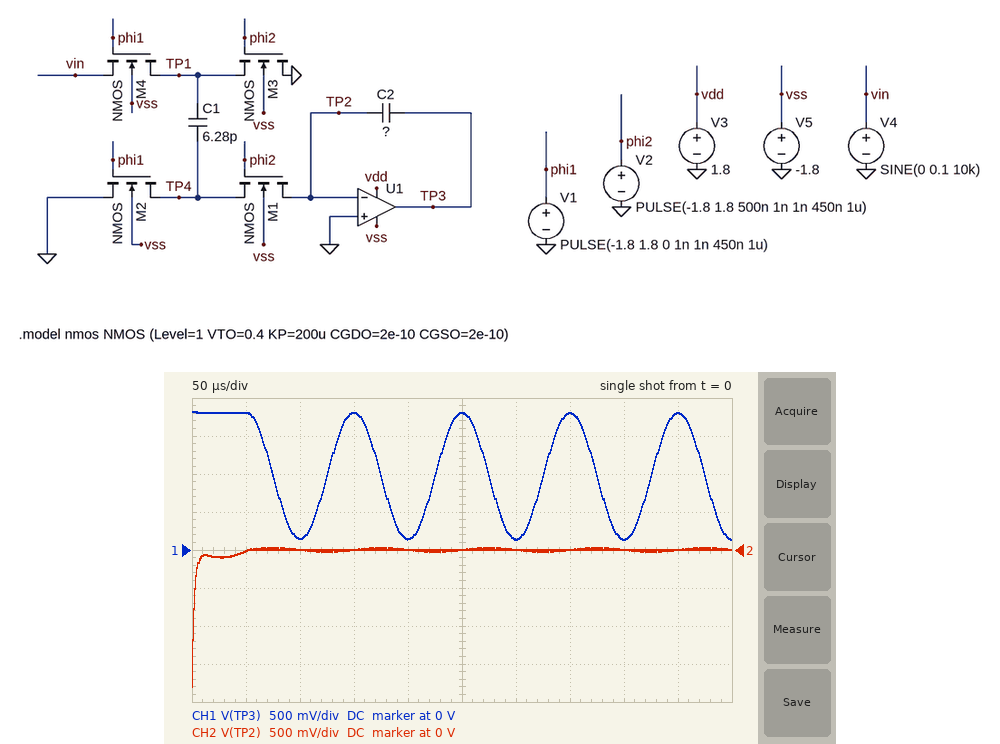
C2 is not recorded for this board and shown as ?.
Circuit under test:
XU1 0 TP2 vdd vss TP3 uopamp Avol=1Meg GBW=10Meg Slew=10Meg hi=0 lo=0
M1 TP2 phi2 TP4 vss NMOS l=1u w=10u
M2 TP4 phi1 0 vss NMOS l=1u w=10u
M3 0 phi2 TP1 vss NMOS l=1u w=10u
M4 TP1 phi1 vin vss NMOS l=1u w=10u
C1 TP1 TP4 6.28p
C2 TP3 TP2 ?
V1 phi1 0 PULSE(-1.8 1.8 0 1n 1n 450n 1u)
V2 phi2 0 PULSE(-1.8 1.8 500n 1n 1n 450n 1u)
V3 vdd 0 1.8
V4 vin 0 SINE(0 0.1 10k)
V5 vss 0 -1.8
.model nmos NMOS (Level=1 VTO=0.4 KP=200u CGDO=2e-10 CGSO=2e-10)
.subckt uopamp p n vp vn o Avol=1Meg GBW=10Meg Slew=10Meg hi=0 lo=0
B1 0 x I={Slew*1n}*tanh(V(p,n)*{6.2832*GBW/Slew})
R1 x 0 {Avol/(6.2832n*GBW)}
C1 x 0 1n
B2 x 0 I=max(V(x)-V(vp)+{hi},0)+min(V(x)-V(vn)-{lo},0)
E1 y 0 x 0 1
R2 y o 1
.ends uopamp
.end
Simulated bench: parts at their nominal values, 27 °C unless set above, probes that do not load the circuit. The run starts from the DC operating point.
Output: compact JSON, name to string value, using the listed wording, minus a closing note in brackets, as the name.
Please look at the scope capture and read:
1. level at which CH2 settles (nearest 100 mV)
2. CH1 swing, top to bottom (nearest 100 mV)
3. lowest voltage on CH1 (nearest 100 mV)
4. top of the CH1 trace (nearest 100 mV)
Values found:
{"level at which CH2 settles": "0 V", "CH1 swing, top to bottom": "1.7 V", "lowest voltage on CH1": "100 mV", "top of the CH1 trace": "1.8 V"}
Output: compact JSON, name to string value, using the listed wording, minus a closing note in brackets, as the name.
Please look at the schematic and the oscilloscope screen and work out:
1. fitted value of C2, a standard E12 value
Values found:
{"fitted value of C2, a standard E12 value": "12 pF"}
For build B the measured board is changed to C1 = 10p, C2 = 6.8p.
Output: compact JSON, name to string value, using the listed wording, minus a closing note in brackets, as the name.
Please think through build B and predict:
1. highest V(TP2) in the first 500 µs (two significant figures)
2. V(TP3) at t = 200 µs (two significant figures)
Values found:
{"highest V(TP2) in the first 500 µs": "71 mV", "V(TP3) at t = 200 µs": "-1.8 V"}
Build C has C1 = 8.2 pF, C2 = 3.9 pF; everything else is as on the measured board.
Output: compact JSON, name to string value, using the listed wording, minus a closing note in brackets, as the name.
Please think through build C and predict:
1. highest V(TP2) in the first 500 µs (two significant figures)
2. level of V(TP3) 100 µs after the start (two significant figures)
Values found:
{"highest V(TP2) in the first 500 µs": "95 mV", "level of V(TP3) 100 µs after the start": "-1.8 V"}
